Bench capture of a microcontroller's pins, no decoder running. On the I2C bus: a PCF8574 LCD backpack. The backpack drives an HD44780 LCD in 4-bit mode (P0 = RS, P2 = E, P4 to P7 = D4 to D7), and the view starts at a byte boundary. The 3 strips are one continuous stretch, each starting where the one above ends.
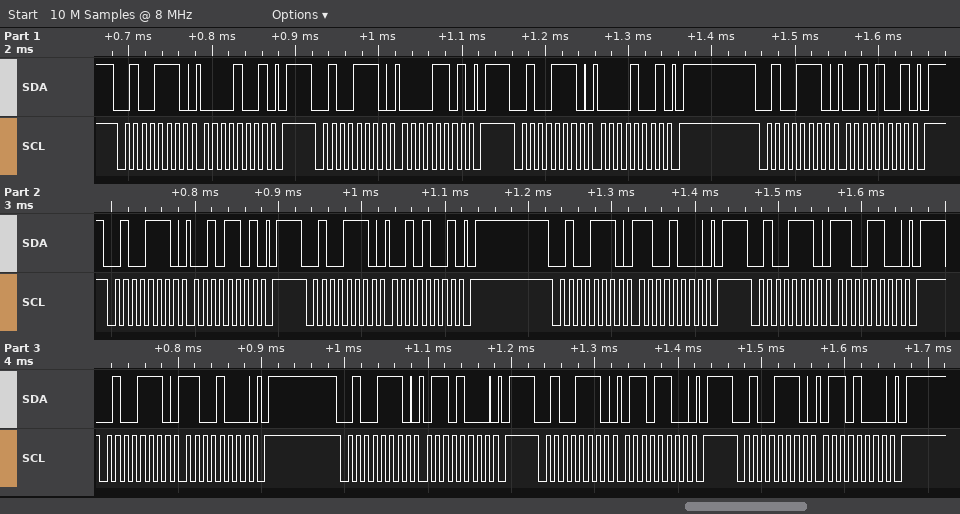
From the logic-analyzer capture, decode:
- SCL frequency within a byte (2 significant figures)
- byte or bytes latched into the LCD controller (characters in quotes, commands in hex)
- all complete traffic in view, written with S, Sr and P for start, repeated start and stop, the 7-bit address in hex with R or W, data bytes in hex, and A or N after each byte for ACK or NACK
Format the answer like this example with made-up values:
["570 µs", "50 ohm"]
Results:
["100 kHz", "data 0x02 0xC6", "S 27W A 09 A P S 27W A 0D A P S 27W A 09 A P S 27W A 29 A P S 27W A 2D A P S 27W A 29 A P S 27W A C8 A P S 27W A CC A P S 27W A C8 A P S 27W A 68 A P S 27W A 6C A P S 27W A 68 A P"]
